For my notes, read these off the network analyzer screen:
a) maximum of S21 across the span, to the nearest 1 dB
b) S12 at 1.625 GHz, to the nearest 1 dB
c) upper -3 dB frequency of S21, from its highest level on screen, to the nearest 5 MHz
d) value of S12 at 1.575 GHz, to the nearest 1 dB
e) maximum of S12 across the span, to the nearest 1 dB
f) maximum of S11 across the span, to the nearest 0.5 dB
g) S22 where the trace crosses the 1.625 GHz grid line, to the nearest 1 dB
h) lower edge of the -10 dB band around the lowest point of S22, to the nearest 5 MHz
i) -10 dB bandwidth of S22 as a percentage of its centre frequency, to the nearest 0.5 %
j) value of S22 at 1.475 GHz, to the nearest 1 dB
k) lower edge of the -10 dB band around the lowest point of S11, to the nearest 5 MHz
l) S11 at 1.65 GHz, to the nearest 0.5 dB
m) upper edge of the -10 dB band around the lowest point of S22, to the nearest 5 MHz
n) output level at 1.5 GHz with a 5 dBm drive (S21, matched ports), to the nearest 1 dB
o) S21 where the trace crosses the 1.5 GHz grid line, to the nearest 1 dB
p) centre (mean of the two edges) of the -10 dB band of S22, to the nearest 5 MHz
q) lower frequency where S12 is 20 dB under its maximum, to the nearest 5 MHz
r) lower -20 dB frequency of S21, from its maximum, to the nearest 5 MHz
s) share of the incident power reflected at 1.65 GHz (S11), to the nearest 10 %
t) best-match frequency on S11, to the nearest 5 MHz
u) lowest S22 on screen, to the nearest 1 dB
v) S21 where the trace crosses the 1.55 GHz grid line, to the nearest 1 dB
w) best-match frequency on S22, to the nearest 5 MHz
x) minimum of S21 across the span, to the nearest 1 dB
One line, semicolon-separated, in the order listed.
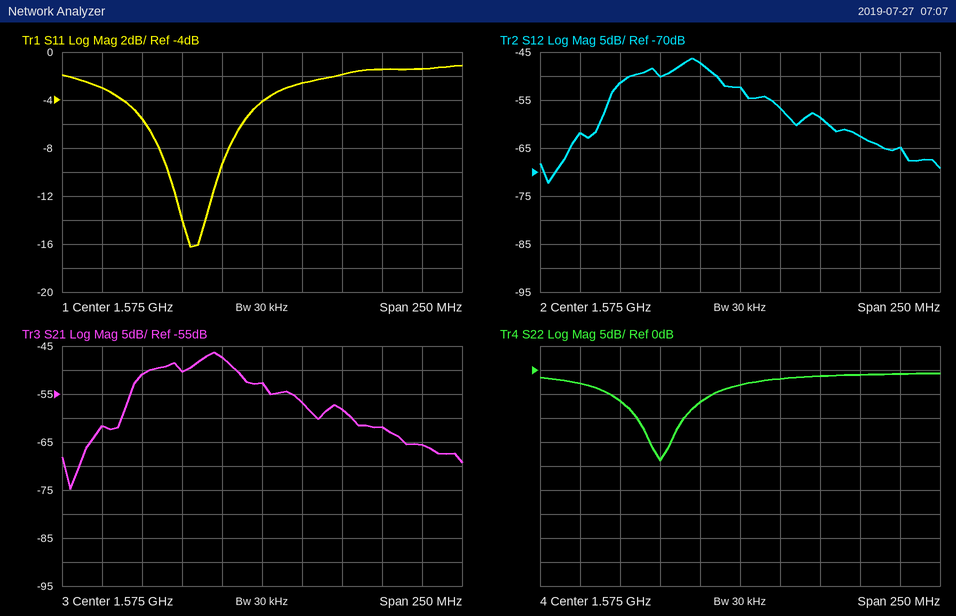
-46 dB; -59 dB; 1.555 GHz; -52 dB; -46 dB; -1.0 dB; -1 dB; 1.510 GHz; 2.0 %; -3 dB; 1.515 GHz; -1.5 dB; 1.540 GHz; -46 dBm; -51 dB; 1.525 GHz; 1.465 GHz; 1.465 GHz; 70 %; 1.530 GHz; -19 dB; -47 dB; 1.525 GHz; -75 dB
